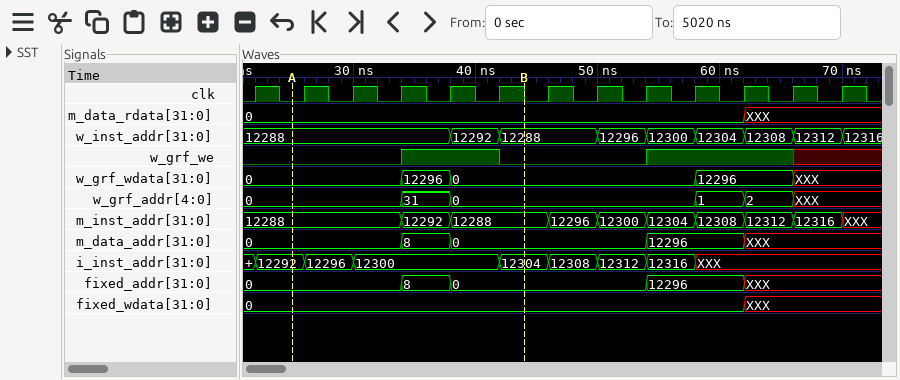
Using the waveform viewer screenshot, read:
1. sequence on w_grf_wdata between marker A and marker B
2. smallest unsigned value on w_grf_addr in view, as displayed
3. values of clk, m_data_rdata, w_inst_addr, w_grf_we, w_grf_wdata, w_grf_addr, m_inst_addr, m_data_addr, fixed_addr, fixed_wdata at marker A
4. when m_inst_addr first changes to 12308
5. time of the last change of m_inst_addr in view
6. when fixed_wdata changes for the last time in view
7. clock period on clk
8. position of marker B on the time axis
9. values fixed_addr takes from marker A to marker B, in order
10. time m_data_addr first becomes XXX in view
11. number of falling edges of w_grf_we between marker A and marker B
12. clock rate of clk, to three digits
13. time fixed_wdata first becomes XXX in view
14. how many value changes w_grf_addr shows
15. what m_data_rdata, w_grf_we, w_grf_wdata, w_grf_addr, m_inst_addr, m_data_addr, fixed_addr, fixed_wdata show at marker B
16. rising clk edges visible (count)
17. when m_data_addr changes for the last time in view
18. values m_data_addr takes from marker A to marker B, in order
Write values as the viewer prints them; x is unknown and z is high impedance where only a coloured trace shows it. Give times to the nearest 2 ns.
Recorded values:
0, 12296, 0
0
clk=0, m_data_rdata=0, w_inst_addr=12288, w_grf_we=0, w_grf_wdata=0, w_grf_addr=0, m_inst_addr=12288, m_data_addr=0, fixed_addr=0, fixed_wdata=0
58 ns
70 ns
62 ns
4 ns
44 ns
0, 8, 0
62 ns
1
250 MHz
62 ns
5
m_data_rdata=0, w_grf_we=0, w_grf_wdata=0, w_grf_addr=0, m_inst_addr=12288, m_data_addr=0, fixed_addr=0, fixed_wdata=0
13
62 ns
0, 8, 0
